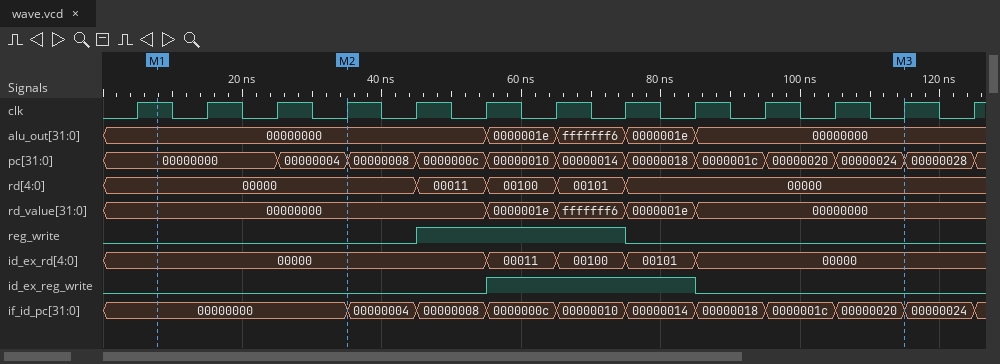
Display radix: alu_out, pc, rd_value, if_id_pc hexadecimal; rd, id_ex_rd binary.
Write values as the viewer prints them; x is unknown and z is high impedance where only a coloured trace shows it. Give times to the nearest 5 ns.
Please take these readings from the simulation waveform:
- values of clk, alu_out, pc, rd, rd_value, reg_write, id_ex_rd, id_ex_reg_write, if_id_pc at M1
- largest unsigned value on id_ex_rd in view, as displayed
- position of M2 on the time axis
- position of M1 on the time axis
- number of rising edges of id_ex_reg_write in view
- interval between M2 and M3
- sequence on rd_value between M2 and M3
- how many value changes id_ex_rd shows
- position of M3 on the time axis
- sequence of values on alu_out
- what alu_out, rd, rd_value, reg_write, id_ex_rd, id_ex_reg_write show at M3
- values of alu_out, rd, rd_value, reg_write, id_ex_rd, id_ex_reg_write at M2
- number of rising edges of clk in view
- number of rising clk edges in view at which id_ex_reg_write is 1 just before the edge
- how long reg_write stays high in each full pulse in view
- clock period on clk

clk=1, alu_out=00000000, pc=00000000, rd=00000, rd_value=00000000, reg_write=0, id_ex_rd=00000, id_ex_reg_write=0, if_id_pc=00000000
00101
35 ns
10 ns
1
80 ns
00000000, 0000001e, fffffff6, 0000001e, 00000000
4
115 ns
00000000, 0000001e, fffffff6, 0000001e, 00000000
alu_out=00000000, rd=00000, rd_value=00000000, reg_write=0, id_ex_rd=00000, id_ex_reg_write=0
alu_out=00000000, rd=00000, rd_value=00000000, reg_write=0, id_ex_rd=00000, id_ex_reg_write=0
13
3
30 ns
10 ns
